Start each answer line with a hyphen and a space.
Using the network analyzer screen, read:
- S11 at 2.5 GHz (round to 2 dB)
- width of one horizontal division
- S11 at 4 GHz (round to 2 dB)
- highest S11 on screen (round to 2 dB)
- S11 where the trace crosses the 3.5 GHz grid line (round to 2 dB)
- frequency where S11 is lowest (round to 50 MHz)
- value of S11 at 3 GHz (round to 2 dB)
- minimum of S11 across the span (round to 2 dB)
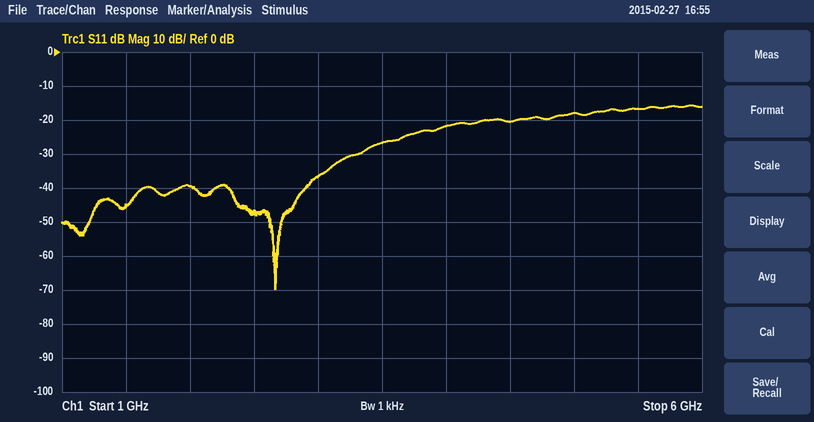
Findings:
- -48 dB
- 500 MHz
- -22 dB
- -16 dB
- -26 dB
- 2.65 GHz
- -36 dB
- -70 dB
